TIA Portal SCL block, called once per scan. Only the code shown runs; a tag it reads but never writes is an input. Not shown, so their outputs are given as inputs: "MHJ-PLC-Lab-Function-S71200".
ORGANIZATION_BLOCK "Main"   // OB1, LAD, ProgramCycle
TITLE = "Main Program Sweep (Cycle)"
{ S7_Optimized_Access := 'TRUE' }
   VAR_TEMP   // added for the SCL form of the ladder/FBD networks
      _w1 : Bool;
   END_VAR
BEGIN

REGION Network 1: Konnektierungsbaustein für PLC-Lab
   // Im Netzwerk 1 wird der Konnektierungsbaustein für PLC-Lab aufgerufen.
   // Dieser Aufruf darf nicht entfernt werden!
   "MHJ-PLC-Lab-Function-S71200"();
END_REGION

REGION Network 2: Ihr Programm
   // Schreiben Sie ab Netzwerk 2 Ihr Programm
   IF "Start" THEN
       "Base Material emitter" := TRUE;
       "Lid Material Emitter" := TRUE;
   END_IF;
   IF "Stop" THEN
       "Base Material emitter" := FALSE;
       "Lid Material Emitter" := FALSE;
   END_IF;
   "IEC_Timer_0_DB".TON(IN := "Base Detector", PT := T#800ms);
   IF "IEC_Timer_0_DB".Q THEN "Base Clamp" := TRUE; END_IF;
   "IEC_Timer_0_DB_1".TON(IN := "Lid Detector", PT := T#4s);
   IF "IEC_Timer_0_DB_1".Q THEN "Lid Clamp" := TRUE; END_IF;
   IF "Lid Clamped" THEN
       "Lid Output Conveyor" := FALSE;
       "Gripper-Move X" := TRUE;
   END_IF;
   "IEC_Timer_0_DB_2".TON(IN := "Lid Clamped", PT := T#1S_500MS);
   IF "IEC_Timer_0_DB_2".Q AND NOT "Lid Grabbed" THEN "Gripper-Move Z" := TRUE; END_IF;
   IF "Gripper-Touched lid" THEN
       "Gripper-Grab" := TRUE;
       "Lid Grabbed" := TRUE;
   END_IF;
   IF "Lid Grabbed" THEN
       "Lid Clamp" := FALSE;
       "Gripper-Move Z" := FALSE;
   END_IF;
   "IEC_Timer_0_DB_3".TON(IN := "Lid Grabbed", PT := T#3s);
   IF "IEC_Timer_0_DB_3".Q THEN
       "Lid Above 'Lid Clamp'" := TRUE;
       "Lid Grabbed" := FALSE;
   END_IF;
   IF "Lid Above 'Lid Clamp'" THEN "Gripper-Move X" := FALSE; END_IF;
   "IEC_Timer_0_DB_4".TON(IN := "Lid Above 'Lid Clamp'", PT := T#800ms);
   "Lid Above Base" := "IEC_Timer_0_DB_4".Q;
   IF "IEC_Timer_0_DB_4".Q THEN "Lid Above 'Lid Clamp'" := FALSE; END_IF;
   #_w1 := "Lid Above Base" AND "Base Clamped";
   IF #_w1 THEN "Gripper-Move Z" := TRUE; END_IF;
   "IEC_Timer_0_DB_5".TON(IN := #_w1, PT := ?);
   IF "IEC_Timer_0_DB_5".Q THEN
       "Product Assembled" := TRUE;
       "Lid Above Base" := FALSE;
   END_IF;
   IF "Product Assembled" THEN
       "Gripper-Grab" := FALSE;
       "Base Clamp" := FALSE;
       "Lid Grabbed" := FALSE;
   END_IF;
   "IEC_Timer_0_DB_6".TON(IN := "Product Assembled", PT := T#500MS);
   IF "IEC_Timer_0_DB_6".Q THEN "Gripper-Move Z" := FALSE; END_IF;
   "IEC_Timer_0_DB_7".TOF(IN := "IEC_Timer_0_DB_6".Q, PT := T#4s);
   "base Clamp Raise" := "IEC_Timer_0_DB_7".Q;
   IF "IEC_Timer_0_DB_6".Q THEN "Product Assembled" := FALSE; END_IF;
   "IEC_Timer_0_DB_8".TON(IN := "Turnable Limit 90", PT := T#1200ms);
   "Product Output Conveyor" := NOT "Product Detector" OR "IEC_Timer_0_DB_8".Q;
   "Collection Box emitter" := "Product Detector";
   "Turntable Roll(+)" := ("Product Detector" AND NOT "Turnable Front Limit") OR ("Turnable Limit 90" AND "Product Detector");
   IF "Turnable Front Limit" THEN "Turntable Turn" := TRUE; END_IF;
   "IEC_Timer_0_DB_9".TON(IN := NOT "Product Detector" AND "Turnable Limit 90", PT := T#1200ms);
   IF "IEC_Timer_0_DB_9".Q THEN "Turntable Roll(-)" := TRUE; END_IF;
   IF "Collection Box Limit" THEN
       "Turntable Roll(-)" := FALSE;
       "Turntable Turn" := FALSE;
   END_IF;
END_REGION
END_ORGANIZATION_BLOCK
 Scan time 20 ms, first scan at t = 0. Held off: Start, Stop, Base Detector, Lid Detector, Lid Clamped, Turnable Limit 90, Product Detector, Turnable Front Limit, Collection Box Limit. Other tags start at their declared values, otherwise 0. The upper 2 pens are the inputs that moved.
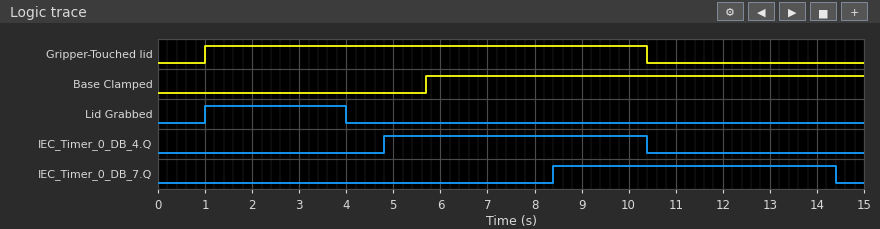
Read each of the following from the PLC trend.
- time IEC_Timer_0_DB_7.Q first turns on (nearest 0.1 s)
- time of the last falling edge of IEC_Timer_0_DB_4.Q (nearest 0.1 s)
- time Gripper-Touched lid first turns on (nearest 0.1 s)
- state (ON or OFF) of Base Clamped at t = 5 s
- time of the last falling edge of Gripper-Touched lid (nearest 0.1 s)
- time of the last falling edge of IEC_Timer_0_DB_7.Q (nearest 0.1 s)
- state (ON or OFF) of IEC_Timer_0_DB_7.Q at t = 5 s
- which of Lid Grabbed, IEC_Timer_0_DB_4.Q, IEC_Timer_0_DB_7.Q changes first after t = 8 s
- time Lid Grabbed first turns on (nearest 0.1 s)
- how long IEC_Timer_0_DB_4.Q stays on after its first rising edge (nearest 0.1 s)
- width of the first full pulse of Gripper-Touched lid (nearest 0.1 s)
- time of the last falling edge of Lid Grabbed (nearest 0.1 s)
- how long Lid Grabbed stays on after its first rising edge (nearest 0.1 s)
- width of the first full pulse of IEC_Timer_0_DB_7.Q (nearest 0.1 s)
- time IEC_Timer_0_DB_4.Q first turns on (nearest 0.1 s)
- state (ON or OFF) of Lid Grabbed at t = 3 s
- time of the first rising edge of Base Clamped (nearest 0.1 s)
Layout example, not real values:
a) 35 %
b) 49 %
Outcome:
a) 8.4 s
b) 10.4 s
c) 1.0 s
d) OFF
e) 10.4 s
f) 14.4 s
g) OFF
h) IEC_Timer_0_DB_7.Q
i) 1.0 s
j) 5.6 s
k) 9.4 s
l) 4.0 s
m) 3.0 s
n) 6.0 s
o) 4.8 s
p) ON
q) 5.7 s
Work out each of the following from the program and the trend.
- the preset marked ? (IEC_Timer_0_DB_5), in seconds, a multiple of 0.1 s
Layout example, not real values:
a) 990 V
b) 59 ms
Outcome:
a) 2.2 s
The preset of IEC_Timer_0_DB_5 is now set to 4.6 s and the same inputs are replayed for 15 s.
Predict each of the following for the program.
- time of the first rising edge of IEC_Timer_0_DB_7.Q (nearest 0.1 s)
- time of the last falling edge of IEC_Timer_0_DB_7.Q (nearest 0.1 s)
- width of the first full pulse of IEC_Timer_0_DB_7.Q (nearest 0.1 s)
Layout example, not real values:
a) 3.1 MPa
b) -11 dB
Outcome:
a) 10.8 s
b) 14.8 s
c) 4.0 s
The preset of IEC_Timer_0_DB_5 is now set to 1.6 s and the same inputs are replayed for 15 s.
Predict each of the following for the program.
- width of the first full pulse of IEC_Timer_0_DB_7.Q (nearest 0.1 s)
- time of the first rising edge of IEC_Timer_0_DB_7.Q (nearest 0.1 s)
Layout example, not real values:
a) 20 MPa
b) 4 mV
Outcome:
a) 6.6 s
b) 7.8 s
